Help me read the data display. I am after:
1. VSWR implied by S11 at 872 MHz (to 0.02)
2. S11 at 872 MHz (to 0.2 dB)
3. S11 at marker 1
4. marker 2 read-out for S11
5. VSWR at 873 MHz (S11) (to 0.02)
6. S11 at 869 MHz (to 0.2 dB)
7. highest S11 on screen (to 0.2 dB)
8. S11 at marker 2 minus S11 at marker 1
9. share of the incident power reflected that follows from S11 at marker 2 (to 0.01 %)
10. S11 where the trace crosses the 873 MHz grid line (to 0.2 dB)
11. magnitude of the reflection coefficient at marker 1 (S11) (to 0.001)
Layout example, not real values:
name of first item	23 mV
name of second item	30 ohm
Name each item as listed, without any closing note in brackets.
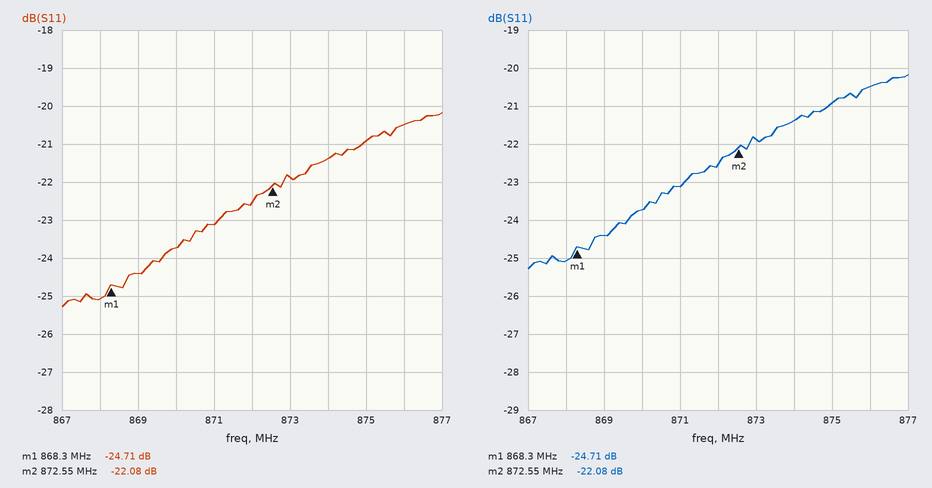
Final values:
VSWR implied by S11 at 872 MHz	1.16
S11 at 872 MHz	-22.6 dB
S11 at marker 1	-24.71 dB
marker 2 read-out for S11	-22.08 dB
VSWR at 873 MHz (S11)	1.18
S11 at 869 MHz	-24.4 dB
highest S11 on screen	-20.2 dB
S11 at marker 2 minus S11 at marker 1	2.63 dB
share of the incident power reflected that follows from S11 at marker 2	0.62 %
S11 where the trace crosses the 873 MHz grid line	-21.8 dB
magnitude of the reflection coefficient at marker 1 (S11)	0.058
